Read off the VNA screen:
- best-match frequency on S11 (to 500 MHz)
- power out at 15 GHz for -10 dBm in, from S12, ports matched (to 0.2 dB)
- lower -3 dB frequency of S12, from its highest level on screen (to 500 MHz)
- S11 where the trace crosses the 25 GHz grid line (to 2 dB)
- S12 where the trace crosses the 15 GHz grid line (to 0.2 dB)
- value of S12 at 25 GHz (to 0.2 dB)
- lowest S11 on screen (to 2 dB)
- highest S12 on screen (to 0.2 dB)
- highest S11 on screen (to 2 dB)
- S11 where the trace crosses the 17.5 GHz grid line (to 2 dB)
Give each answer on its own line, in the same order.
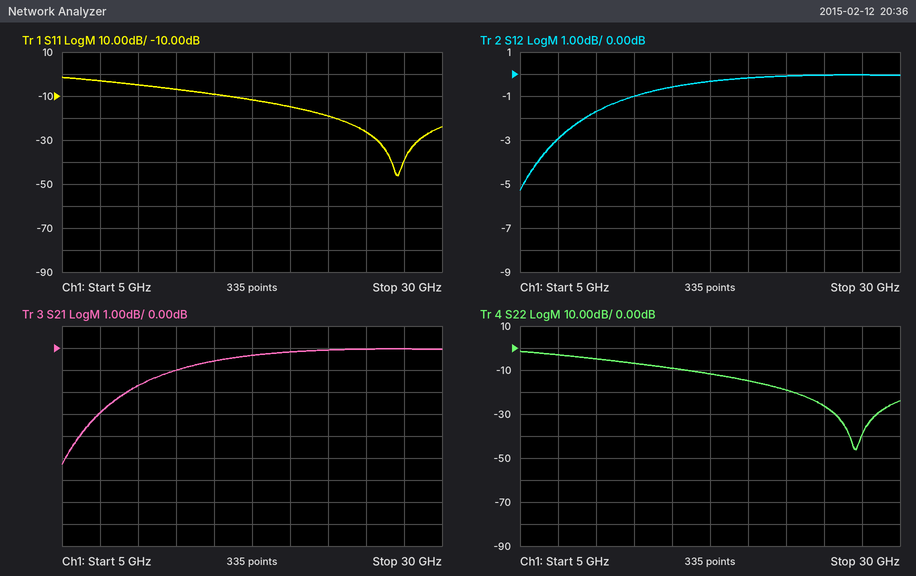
27.0 GHz
-10.6 dBm
7.5 GHz
-26 dB
-0.6 dB
0.0 dB
-46 dB
0.0 dB
-2 dB
-12 dB
